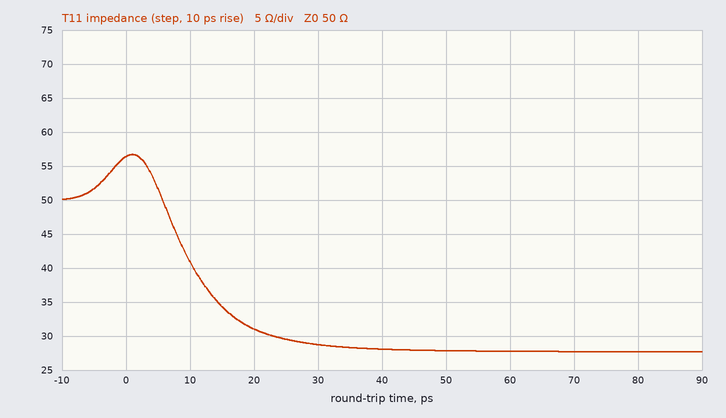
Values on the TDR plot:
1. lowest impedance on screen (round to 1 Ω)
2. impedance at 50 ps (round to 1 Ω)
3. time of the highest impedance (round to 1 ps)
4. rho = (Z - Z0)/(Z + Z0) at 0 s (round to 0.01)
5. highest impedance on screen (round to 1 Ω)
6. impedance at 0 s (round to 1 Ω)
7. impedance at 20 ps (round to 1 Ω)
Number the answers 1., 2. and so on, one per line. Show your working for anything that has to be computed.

1. 28 Ω
2. 28 Ω
3. 1 ps
4. (56 − 50)/(56 + 50) ≈ +0.06
5. 57 Ω
6. 56 Ω
7. 31 Ω
